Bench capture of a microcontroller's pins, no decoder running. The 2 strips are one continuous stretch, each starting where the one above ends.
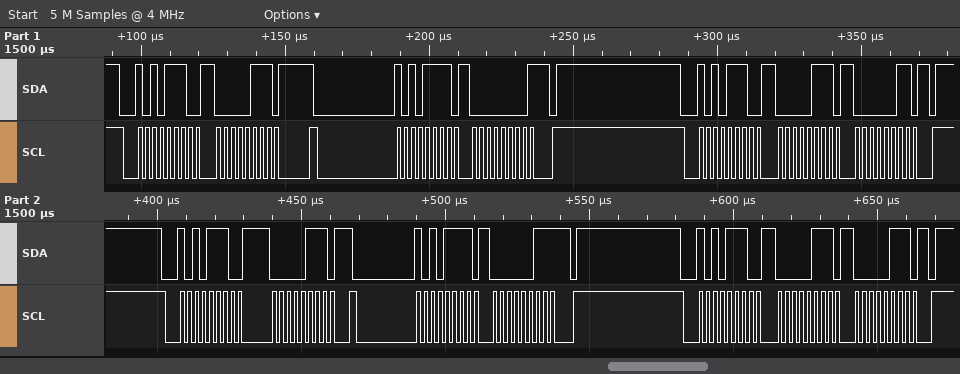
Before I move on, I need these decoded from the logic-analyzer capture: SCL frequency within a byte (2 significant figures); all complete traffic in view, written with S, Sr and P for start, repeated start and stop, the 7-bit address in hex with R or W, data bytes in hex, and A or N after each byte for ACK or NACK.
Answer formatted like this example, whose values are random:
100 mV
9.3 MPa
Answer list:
400 kHz
S 57W A 07 A Sr 57R A 00 N P S 57W A 07 A 03 A P S 57W A 07 A Sr 57R A 03 N P S 57W A 07 A 07 A P
